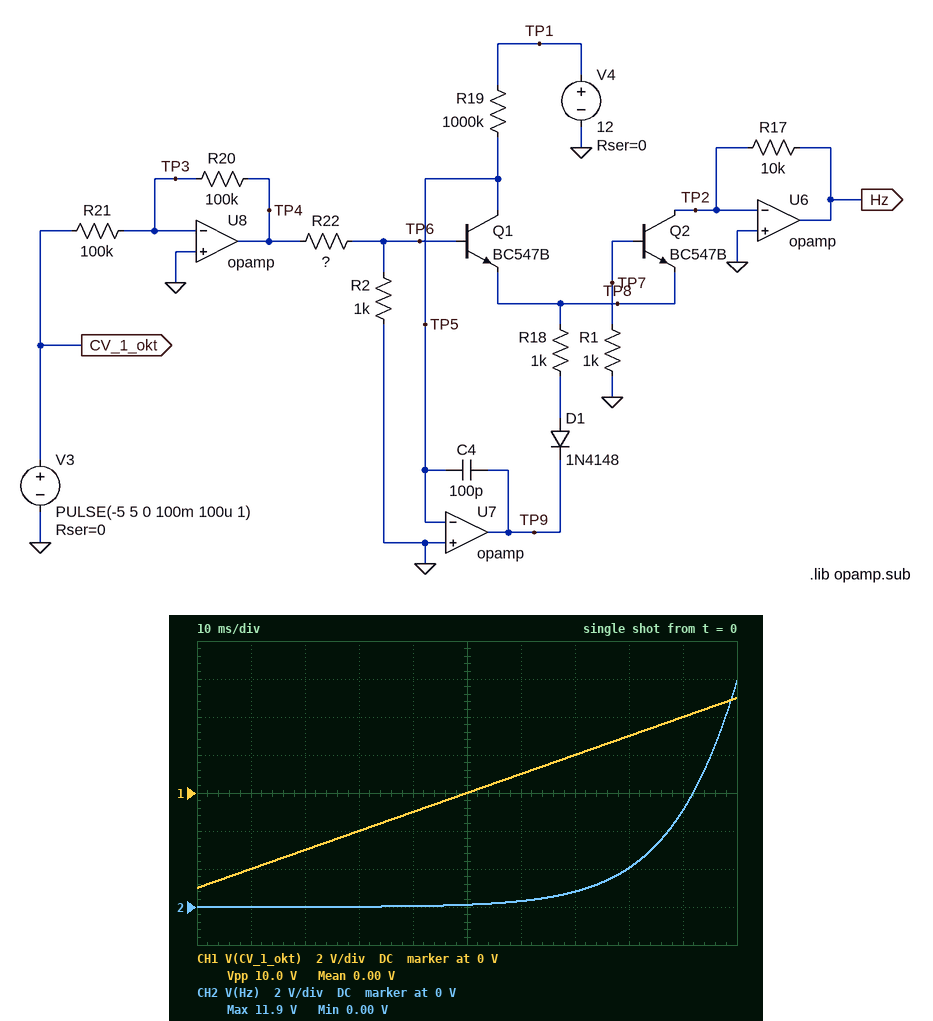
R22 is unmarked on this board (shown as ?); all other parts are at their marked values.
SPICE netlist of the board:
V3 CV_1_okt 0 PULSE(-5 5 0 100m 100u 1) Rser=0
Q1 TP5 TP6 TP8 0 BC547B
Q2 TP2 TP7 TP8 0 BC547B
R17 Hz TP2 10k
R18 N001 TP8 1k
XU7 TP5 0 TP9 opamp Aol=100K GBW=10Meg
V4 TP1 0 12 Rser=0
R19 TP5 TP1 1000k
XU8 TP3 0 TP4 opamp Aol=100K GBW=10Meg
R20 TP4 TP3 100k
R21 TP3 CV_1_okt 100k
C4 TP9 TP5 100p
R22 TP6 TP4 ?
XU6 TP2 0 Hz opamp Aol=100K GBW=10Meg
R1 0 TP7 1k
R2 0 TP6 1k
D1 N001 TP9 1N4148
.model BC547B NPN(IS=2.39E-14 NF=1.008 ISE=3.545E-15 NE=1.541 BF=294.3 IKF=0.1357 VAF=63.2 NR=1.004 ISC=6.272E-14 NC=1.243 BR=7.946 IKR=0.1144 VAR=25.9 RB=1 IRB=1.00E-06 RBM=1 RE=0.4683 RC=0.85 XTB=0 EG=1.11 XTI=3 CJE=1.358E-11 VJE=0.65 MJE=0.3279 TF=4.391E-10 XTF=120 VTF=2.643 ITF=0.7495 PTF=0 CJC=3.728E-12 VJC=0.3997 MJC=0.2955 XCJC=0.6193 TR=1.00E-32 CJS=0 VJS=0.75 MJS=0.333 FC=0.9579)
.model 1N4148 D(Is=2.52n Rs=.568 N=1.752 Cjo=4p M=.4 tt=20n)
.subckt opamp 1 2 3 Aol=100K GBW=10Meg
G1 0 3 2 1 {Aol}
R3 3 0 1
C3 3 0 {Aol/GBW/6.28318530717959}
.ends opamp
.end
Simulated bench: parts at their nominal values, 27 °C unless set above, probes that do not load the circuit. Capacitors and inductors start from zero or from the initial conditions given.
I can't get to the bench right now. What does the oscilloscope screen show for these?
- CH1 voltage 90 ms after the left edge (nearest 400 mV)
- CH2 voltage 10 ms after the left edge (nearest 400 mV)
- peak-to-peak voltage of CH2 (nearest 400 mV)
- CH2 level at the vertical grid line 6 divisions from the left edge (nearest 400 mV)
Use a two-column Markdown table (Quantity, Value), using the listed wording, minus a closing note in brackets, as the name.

| Quantity | Value |
|---|---|
| CH1 voltage 90 ms after the left edge | 4.0 V |
| CH2 voltage 10 ms after the left edge | 0 V |
| peak-to-peak voltage of CH2 | 12.0 V |
| CH2 level at the vertical grid line 6 divisions from the left edge | 400 mV |
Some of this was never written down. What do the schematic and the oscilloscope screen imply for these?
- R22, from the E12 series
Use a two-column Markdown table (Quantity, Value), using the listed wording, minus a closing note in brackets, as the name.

| Quantity | Value |
|---|---|
| R22, from the E12 series | 39 kΩ |
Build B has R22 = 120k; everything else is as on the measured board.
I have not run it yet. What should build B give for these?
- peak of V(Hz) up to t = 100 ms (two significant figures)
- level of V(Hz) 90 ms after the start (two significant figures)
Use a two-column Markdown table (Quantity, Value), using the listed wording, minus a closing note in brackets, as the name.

| Quantity | Value |
|---|---|
| peak of V(Hz) up to t = 100 ms | 580 mV |
| level of V(Hz) 90 ms after the start | 420 mV |
